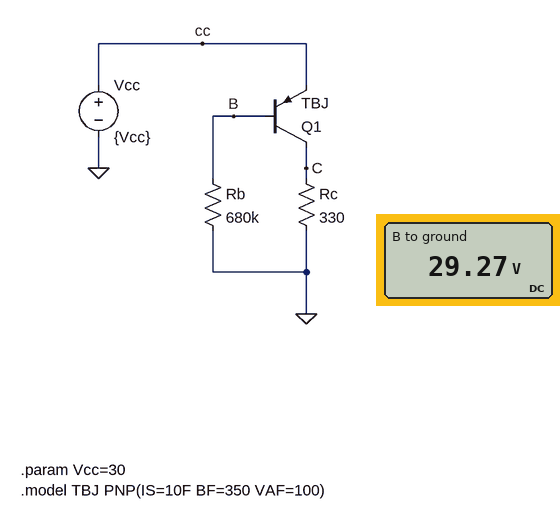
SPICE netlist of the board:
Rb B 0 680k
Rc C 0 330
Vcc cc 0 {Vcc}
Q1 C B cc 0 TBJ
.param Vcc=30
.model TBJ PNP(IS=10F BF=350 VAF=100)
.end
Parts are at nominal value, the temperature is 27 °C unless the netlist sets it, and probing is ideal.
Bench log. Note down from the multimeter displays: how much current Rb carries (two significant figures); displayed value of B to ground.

43 µA
29.27 V
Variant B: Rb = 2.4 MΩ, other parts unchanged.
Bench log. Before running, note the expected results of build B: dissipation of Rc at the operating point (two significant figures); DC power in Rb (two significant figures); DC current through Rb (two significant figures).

9.8 mW
360 µW
12 µA
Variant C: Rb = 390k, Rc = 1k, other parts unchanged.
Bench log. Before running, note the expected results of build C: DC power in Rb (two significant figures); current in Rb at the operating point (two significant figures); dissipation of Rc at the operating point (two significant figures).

2.2 mW
75 µA
720 mW
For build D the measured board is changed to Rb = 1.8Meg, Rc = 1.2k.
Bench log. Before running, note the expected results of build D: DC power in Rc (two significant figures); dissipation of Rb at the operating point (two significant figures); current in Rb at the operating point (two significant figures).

57 mW
480 µW
16 µA
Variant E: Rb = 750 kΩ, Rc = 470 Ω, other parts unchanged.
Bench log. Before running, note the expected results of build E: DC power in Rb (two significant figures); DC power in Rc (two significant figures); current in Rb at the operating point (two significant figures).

1.1 mW
130 mW
39 µA
